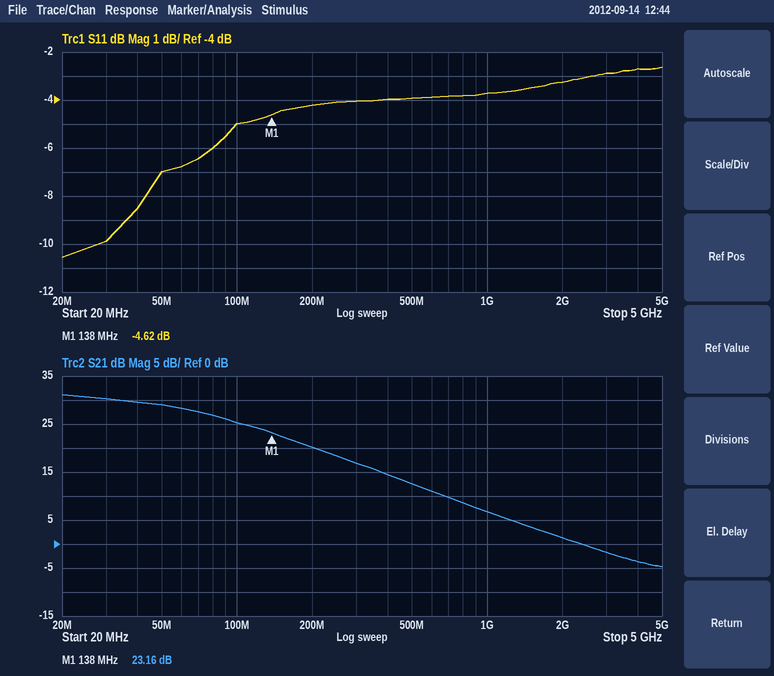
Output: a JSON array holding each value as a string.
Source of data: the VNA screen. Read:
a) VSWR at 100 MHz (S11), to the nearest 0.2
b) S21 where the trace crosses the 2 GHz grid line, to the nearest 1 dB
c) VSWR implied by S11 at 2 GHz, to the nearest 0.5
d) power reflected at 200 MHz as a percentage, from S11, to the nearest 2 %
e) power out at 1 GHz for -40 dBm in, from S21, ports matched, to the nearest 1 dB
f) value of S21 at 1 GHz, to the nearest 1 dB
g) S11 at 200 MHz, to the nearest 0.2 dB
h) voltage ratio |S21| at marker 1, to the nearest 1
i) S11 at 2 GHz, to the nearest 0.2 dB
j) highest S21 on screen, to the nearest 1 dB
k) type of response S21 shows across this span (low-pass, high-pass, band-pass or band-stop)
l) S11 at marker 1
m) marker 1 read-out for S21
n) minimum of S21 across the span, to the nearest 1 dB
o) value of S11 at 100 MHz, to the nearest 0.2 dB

["3.6", "1 dB", "5.5", "38 %", "-33 dBm", "7 dB", "-4.2 dB", "14", "-3.2 dB", "31 dB", "low-pass", "-4.62 dB", "23.16 dB", "-5 dB", "-5.0 dB"]
